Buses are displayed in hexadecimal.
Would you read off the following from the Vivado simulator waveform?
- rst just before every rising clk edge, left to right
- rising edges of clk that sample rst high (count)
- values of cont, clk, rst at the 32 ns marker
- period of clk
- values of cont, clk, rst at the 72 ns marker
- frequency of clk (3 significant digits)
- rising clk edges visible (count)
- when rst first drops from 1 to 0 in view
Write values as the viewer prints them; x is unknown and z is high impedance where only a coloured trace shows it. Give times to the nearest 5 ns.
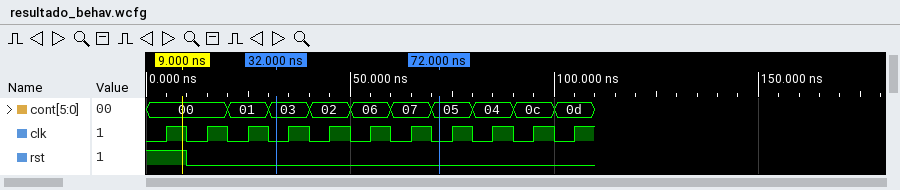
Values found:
1 0 0 0 0 0 0 0 0 0 0
1
cont=03, clk=0, rst=0
10 ns
cont=05, clk=0, rst=0
100 MHz
11
10 ns
